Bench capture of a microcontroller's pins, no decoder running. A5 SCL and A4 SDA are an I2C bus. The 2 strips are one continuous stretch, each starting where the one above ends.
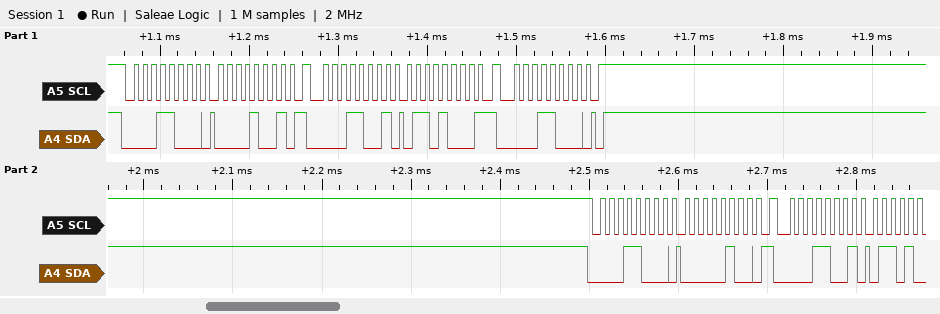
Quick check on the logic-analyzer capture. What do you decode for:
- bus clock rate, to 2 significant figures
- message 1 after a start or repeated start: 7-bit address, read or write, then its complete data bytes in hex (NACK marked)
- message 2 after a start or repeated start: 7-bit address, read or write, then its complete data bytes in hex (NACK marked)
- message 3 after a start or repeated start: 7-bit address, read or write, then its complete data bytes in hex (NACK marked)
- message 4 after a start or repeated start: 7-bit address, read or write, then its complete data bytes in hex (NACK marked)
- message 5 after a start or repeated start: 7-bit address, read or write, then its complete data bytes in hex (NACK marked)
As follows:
100 kHz
0x0C write: 09
0x0C read: 68 NACK
0x0C write
0x0C write: 04
0x0C read
